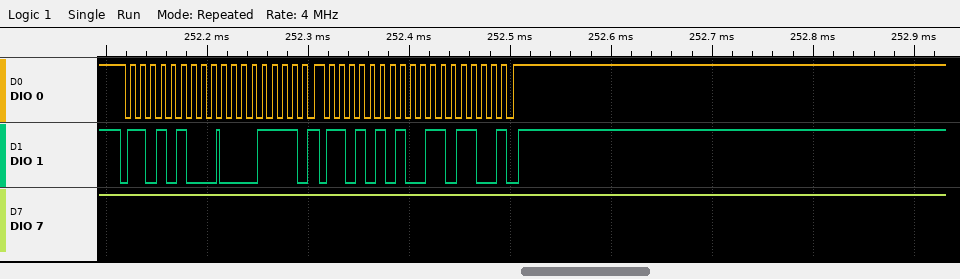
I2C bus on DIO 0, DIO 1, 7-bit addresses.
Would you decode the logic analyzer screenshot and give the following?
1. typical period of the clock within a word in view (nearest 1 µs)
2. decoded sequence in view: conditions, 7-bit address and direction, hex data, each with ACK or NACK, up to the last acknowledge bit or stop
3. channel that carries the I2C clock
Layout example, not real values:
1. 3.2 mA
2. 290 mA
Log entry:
1. 10 µs
2. start, address 6A write ACK, 0F ACK, repeated start, address 6A read ACK, 6C NACK, stop
3. DIO 0
